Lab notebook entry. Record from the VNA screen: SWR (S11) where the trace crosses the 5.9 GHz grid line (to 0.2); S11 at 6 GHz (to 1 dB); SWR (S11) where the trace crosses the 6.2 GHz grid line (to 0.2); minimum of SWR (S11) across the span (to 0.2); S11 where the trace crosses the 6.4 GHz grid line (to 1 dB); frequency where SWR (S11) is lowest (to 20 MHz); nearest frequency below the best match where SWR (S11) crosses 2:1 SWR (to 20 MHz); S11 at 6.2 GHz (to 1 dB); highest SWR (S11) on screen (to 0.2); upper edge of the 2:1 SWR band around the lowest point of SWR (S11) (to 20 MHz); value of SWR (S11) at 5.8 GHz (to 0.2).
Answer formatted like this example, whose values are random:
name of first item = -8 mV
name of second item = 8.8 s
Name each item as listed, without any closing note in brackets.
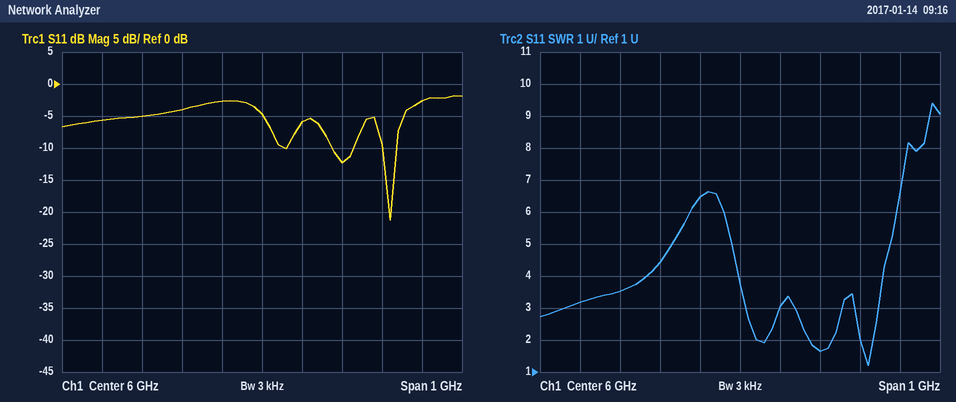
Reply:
SWR (S11) where the trace crosses the 5.9 GHz grid line = 6.4
S11 at 6 GHz = -5 dB
SWR (S11) where the trace crosses the 6.2 GHz grid line = 1.6
minimum of SWR (S11) across the span = 1.2
S11 where the trace crosses the 6.4 GHz grid line = -3 dB
frequency where SWR (S11) is lowest = 6.32 GHz
nearest frequency below the best match where SWR (S11) crosses 2:1 SWR = 6.30 GHz
S11 at 6.2 GHz = -12 dB
highest SWR (S11) on screen = 9.4
upper edge of the 2:1 SWR band around the lowest point of SWR (S11) = 6.34 GHz
value of SWR (S11) at 5.8 GHz = 4.4
